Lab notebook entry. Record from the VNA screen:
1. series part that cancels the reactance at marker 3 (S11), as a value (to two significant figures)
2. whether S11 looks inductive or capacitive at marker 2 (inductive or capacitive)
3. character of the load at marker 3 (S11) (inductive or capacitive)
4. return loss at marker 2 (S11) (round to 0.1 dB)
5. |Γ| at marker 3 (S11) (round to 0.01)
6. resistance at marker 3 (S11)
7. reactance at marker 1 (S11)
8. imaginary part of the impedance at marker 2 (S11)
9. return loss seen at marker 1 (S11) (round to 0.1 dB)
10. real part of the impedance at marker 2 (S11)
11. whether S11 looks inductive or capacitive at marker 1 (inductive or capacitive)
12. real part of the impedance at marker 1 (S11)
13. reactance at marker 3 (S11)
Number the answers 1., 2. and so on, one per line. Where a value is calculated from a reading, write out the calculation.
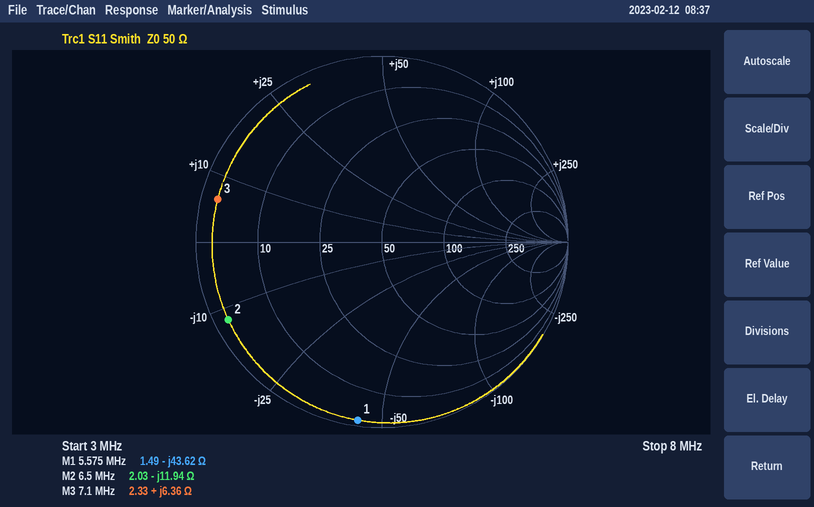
1. C = 1/(2π × 7.1 MHz × 6.36 Ω) ≈ 3.5 nF
2. capacitive
3. inductive
4. 0.7 dB
5. 0.91
6. 2.33 Ω
7. -43.62 Ω
8. -11.94 Ω
9. 0.3 dB
10. 2.03 Ω
11. capacitive
12. 1.49 Ω
13. +6.36 Ω
